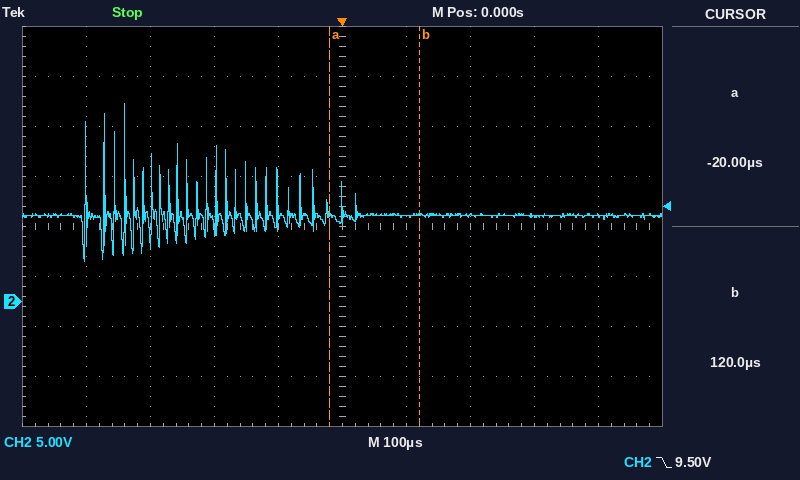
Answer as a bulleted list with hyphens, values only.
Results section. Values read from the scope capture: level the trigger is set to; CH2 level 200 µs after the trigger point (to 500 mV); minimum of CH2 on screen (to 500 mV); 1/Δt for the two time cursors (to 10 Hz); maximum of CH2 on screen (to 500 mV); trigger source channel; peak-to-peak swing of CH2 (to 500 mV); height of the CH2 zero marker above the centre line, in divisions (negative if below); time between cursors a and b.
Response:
- 9.50 V
- 8.5 V
- 4.0 V
- 7.14 kHz
- 20.0 V
- CH2
- 16.0 V
- -1.5 div
- 140 µs
